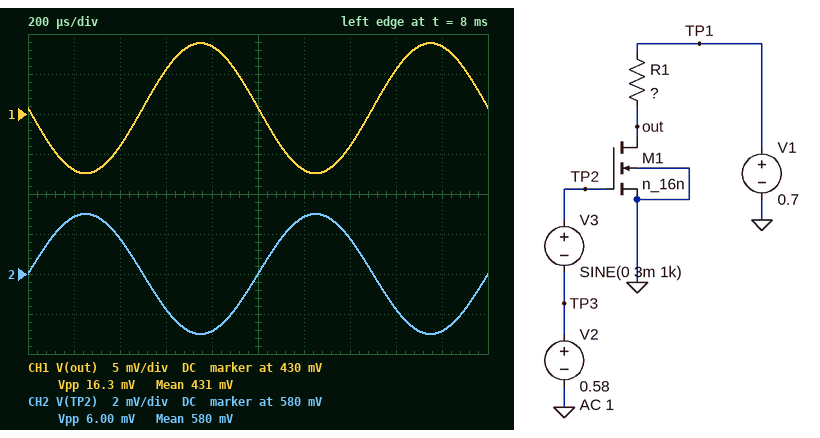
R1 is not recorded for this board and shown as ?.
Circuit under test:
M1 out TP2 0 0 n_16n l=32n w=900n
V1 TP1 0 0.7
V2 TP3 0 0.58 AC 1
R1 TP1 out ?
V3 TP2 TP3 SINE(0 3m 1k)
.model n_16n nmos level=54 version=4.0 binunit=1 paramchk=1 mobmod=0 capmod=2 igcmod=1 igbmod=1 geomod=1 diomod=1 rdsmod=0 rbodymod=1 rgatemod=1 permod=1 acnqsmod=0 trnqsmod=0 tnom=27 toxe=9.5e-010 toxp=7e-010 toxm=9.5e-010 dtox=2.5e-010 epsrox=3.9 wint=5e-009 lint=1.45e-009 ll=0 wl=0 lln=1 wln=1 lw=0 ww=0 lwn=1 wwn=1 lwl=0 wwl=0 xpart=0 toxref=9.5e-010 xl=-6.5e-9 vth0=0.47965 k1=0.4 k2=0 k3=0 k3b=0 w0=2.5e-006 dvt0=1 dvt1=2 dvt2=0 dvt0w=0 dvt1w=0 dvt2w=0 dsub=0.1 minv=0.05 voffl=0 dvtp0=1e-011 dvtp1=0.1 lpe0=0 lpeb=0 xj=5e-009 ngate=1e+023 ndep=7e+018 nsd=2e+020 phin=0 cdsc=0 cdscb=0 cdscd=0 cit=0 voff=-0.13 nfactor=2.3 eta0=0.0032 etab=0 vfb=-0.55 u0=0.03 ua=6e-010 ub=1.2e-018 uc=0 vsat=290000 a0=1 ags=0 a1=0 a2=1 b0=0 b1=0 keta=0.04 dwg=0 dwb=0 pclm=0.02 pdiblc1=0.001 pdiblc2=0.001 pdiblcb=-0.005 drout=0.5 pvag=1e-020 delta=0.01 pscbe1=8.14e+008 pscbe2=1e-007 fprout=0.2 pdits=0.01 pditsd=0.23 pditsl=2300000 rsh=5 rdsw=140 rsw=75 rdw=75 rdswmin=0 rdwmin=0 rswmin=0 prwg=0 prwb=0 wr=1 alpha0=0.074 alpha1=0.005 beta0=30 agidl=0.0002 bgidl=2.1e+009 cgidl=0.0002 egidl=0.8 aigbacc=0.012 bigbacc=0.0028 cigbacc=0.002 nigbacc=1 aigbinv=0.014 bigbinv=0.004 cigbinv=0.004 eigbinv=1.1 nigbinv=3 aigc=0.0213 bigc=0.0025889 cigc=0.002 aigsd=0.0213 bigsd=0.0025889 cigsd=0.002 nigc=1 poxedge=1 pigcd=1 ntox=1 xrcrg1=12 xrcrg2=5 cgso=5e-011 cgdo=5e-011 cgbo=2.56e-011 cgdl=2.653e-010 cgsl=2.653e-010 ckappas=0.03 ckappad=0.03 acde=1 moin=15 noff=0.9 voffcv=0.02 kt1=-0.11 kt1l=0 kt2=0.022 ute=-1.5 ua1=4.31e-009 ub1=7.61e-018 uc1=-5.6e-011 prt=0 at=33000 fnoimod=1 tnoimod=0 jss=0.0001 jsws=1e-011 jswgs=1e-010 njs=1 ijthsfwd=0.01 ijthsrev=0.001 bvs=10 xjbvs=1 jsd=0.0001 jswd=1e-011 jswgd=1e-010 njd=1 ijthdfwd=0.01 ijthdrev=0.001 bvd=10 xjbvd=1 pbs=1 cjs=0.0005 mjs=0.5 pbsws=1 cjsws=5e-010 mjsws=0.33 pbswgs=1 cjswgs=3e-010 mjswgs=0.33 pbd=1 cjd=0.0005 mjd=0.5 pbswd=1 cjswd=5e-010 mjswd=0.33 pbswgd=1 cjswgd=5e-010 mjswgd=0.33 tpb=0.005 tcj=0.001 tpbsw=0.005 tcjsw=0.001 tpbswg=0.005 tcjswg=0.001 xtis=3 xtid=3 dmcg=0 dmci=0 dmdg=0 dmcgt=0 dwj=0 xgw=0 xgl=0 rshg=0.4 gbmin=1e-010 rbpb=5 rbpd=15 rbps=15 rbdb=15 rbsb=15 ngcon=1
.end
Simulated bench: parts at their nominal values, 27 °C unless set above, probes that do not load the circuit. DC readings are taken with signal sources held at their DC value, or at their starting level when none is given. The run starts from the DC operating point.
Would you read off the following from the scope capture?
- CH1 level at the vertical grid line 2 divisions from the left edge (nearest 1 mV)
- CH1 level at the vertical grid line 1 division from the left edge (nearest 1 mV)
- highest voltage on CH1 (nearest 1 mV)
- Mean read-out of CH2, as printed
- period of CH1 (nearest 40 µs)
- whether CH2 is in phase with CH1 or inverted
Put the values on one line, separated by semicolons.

426 mV; 423 mV; 439 mV; 580 mV; 1.00 ms; inverted
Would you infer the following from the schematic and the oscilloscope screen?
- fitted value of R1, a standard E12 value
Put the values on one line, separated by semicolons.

2.7 kΩ
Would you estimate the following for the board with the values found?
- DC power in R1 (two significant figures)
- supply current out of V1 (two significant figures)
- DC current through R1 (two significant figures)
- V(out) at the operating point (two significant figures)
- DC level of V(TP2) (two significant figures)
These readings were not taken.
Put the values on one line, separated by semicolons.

27 µW; 100 µA; 100 µA; 430 mV; 580 mV
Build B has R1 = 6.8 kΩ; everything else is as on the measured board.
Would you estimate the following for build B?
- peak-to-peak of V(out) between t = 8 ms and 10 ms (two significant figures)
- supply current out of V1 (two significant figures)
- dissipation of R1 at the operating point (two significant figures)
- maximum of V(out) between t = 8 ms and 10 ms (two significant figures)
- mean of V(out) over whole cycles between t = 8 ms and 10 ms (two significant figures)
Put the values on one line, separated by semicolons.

16 mV; 83 µA; 47 µW; 140 mV; 130 mV
